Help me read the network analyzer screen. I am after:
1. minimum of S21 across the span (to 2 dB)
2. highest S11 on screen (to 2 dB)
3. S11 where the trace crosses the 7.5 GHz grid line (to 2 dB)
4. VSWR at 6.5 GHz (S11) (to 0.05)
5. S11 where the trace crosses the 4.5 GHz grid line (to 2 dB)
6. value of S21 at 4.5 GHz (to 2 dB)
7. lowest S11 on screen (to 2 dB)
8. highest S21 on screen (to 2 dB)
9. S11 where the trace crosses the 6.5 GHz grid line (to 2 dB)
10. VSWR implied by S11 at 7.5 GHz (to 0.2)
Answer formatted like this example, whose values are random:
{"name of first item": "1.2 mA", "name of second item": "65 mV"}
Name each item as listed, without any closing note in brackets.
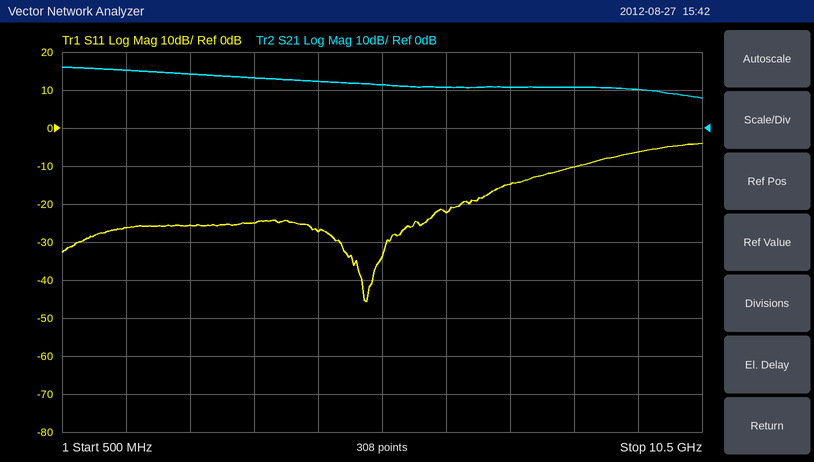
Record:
{"minimum of S21 across the span": "8 dB", "highest S11 on screen": "-4 dB", "S11 where the trace crosses the 7.5 GHz grid line": "-14 dB", "VSWR at 6.5 GHz (S11)": "1.15", "S11 where the trace crosses the 4.5 GHz grid line": "-28 dB", "value of S21 at 4.5 GHz": "12 dB", "lowest S11 on screen": "-46 dB", "highest S21 on screen": "16 dB", "S11 where the trace crosses the 6.5 GHz grid line": "-22 dB", "VSWR implied by S11 at 7.5 GHz": "1.4"}
